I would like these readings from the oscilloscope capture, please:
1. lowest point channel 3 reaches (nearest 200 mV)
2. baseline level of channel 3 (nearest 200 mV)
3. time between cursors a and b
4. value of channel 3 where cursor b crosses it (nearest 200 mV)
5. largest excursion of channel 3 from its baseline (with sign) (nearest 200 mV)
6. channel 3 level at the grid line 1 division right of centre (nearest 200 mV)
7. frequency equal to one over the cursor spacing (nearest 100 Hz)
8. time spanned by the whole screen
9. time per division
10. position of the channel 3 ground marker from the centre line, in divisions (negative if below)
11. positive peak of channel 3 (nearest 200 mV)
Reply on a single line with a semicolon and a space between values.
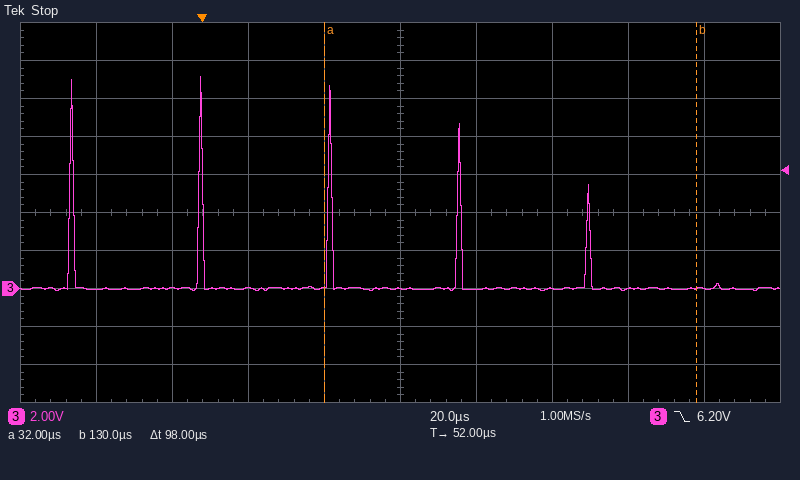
-200 mV; 0.0 V; 98 µs; 0.0 V; +11.2 V; 0.0 V; 10.2 kHz; 200 µs; 20 µs; -2.0 div; 11.2 V
